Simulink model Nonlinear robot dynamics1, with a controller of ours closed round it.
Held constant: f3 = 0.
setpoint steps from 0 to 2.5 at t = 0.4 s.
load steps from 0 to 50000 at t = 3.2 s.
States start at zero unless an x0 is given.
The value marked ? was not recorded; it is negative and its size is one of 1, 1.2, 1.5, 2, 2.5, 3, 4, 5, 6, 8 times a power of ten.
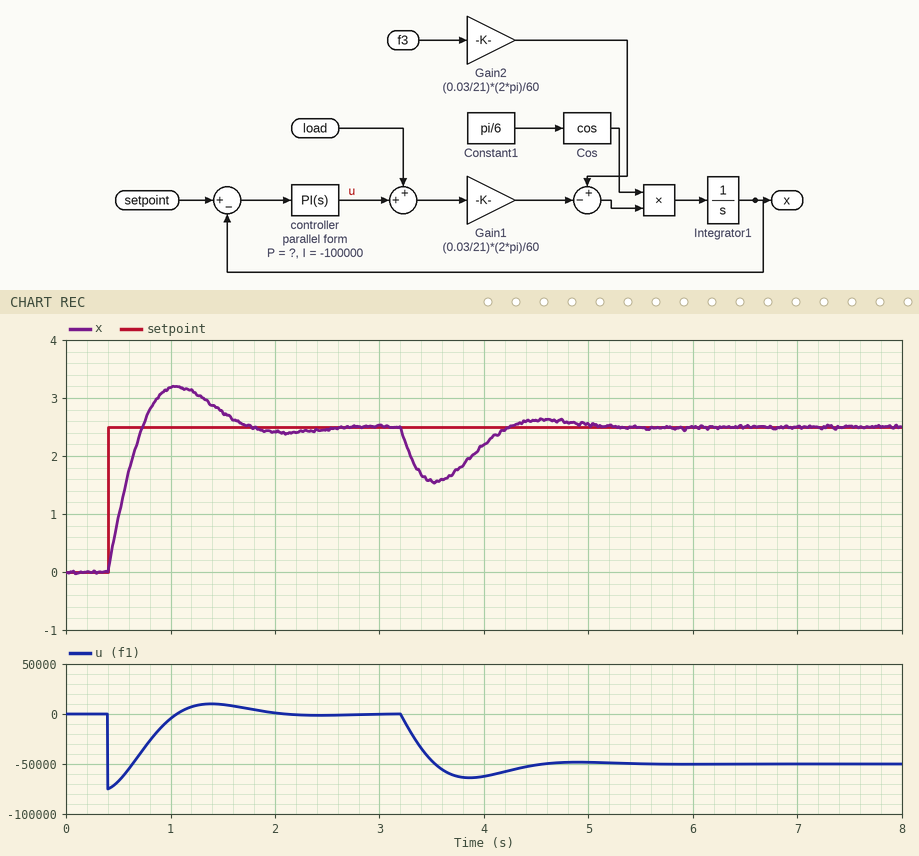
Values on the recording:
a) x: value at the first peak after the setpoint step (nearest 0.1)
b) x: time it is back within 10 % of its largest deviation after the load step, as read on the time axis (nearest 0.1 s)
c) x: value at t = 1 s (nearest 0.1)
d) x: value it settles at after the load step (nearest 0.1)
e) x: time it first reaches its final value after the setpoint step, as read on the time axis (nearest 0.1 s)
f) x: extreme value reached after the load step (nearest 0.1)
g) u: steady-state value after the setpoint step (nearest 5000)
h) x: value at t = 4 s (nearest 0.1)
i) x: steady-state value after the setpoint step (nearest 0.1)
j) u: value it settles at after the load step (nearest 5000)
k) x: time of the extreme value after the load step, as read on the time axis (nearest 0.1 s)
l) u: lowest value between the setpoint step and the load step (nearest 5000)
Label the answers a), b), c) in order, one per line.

a) 3.2
b) 4.8 s
c) 3.2
d) 2.5
e) 0.7 s
f) 1.6
g) 0
h) 2.2
i) 2.5
j) -50000
k) 3.5 s
l) -75000
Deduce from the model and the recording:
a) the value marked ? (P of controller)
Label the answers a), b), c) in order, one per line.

a) -30000
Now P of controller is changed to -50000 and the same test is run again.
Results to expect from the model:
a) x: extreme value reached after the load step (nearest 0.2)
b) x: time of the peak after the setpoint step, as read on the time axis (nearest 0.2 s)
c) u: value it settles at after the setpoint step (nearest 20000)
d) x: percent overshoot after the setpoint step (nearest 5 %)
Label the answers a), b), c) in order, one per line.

a) 1.8
b) 1.0 s
c) 0
d) 15 %
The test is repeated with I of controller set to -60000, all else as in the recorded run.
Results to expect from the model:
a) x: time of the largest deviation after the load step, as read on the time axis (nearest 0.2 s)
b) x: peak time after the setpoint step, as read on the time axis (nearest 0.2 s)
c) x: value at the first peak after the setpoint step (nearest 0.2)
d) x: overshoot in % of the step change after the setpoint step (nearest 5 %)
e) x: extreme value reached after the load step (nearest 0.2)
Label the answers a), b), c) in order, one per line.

a) 3.6 s
b) 1.2 s
c) 3.0
d) 20 %
e) 1.4
